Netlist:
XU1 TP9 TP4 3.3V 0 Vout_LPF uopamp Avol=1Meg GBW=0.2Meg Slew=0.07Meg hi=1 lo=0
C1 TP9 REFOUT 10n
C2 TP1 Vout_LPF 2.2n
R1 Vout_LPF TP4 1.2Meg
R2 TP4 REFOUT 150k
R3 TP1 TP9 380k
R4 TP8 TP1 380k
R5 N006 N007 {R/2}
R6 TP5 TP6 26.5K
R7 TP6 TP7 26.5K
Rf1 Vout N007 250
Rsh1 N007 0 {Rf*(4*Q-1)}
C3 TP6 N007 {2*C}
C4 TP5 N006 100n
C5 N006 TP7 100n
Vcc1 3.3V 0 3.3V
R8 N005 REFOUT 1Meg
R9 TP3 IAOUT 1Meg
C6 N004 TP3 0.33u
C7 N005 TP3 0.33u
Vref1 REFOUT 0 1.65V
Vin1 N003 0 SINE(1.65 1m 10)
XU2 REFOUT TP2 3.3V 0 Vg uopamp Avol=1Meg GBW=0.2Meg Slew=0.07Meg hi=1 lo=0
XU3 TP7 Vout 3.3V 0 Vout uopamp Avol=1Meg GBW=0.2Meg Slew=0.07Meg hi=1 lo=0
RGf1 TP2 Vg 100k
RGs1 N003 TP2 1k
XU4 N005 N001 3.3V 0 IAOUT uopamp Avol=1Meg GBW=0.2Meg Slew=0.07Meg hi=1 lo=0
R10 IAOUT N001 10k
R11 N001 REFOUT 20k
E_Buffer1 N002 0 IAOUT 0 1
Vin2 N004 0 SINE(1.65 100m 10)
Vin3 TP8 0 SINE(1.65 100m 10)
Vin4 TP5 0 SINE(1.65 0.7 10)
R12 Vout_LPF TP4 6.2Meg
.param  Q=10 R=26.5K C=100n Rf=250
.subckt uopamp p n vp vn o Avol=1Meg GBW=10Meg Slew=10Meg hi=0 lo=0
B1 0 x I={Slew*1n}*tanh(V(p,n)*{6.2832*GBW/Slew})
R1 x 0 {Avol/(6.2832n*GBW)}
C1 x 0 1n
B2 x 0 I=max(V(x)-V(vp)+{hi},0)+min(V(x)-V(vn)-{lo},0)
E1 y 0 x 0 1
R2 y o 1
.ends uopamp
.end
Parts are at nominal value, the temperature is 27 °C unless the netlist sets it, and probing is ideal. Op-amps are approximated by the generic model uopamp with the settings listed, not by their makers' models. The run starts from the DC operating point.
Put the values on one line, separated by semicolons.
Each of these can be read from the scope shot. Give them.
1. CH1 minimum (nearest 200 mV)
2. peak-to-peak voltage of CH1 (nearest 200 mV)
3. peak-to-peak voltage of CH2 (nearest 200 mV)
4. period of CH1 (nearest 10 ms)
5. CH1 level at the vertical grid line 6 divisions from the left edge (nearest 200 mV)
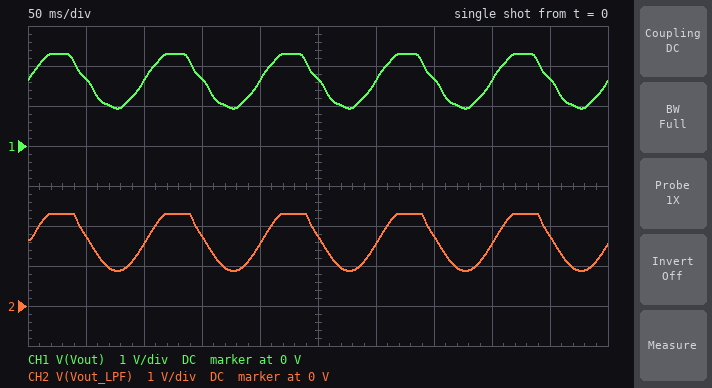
1.0 V; 1.4 V; 1.4 V; 100 ms; 1.6 V
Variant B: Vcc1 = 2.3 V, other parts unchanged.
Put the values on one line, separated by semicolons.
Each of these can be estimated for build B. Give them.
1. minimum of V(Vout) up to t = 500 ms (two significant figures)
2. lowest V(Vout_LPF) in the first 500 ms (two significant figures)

710 mV; 860 mV
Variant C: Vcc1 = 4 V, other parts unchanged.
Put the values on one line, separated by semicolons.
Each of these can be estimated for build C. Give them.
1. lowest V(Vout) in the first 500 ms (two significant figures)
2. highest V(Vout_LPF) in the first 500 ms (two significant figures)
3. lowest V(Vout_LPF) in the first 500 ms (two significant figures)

950 mV; 2.4 V; 880 mV
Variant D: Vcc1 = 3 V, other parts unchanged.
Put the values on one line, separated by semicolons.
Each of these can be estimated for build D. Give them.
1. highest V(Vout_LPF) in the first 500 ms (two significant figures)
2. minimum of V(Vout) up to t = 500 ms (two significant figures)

2.0 V; 780 mV
